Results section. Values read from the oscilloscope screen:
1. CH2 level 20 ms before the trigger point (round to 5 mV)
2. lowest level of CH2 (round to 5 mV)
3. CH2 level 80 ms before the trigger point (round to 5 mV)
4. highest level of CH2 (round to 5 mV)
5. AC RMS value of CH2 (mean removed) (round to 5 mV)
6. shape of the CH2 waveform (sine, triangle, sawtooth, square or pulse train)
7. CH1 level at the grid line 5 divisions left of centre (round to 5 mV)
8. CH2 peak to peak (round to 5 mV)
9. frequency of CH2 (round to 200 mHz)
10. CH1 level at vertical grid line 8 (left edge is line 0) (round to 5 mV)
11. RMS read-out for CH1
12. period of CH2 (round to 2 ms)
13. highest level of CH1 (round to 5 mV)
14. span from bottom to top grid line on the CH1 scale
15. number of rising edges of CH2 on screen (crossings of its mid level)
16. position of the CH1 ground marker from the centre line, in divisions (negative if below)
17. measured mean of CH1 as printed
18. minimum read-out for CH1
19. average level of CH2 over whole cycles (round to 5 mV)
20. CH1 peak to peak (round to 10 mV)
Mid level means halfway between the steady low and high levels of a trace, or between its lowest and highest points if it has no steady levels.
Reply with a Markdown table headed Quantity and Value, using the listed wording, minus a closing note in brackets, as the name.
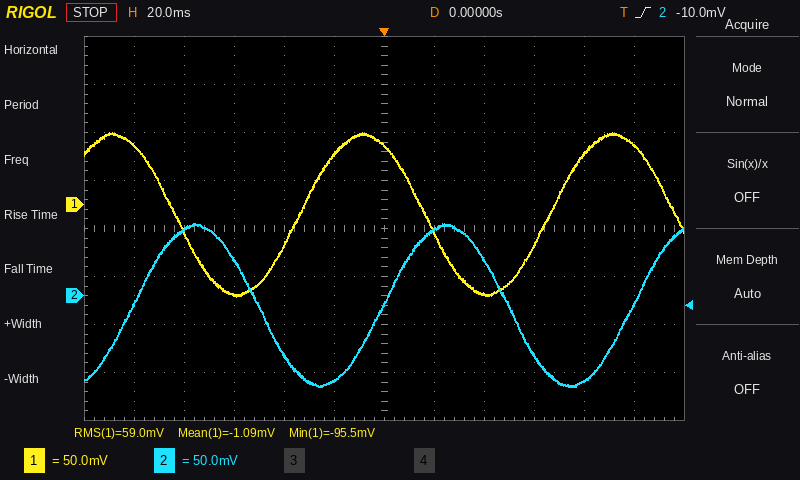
| Quantity | Value |
|---|---|
| CH2 level 20 ms before the trigger point | -90 mV |
| lowest level of CH2 | -95 mV |
| CH2 level 80 ms before the trigger point | 70 mV |
| highest level of CH2 | 75 mV |
| AC RMS value of CH2 (mean removed) | 60 mV |
| shape of the CH2 waveform | sine |
| CH1 level at the grid line 5 divisions left of centre | 60 mV |
| CH2 peak to peak | 170 mV |
| frequency of CH2 | 10.0 Hz |
| CH1 level at vertical grid line 8 (left edge is line 0) | -95 mV |
| RMS read-out for CH1 | 59.0 mV |
| period of CH2 | 100 ms |
| highest level of CH1 | 75 mV |
| span from bottom to top grid line on the CH1 scale | 400 mV |
| number of rising edges of CH2 on screen | 3 |
| position of the CH1 ground marker from the centre line, in divisions | +0.5 div |
| measured mean of CH1 as printed | -1.09 mV |
| minimum read-out for CH1 | -95.5 mV |
| average level of CH2 over whole cycles | -10 mV |
| CH1 peak to peak | 170 mV |
